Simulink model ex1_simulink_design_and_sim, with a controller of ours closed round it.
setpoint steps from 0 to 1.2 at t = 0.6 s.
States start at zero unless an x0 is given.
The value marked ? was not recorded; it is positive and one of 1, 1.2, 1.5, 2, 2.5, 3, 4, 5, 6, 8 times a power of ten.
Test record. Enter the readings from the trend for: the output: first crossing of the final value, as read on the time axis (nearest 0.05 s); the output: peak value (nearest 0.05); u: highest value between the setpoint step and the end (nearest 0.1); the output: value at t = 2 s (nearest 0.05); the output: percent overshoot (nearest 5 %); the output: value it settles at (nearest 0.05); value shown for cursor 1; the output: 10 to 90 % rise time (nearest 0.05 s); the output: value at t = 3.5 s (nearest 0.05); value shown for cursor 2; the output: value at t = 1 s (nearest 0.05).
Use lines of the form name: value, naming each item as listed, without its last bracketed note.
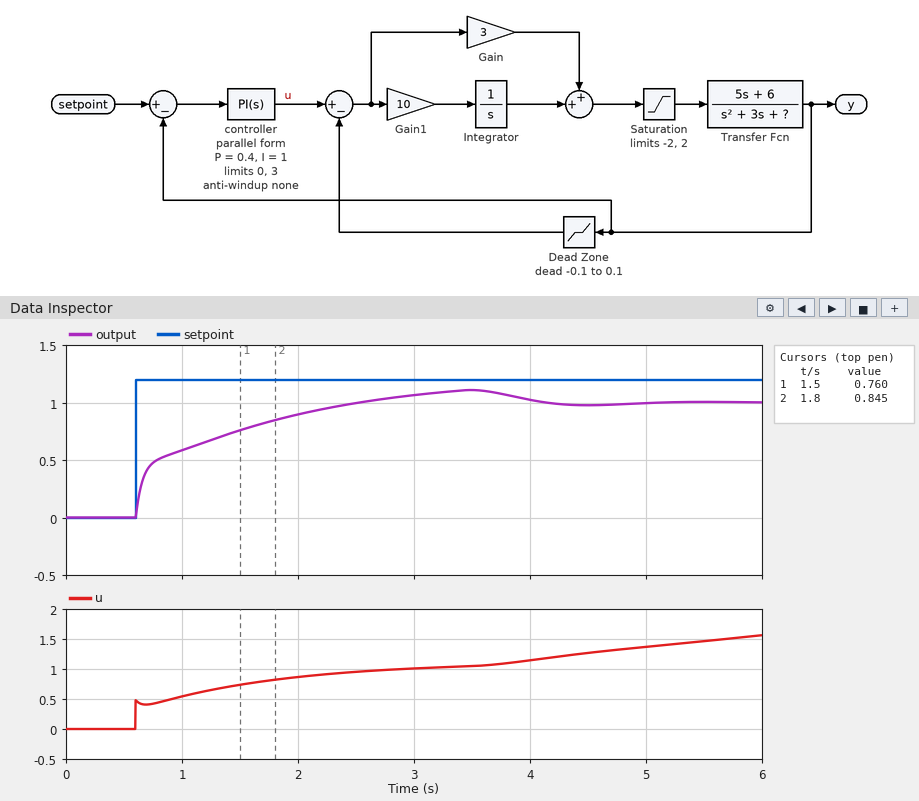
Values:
the output: first crossing of the final value, as read on the time axis: 2.55 s
the output: peak value: 1.10
u: highest value between the setpoint step and the end: 1.6
the output: value at t = 2 s: 0.90
the output: percent overshoot: 10 %
the output: value it settles at: 1.00
value shown for cursor 1: 0.760
the output: 10 to 90 % rise time: 1.40 s
the output: value at t = 3.5 s: 1.10
value shown for cursor 2: 0.845
the output: value at t = 1 s: 0.60
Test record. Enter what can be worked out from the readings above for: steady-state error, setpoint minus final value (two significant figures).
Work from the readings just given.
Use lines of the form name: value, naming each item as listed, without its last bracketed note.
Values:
steady-state error, setpoint minus final value: 0.20
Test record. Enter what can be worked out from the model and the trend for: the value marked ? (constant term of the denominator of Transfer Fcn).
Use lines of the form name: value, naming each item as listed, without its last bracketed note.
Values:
the value marked ?: 12
